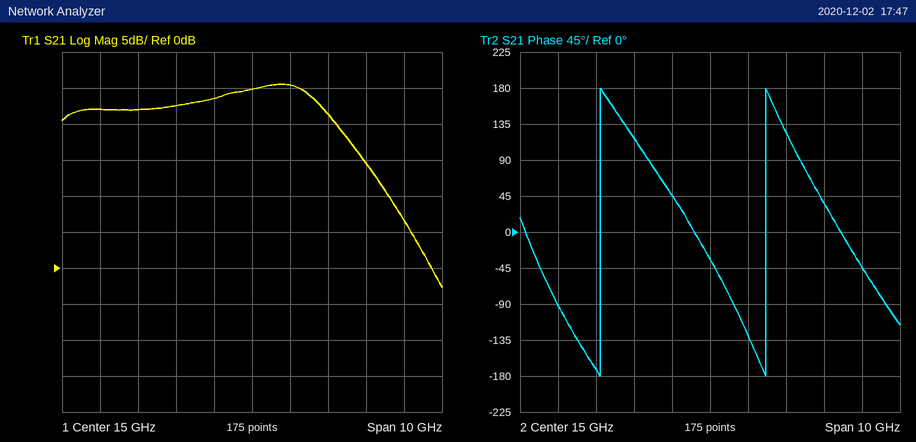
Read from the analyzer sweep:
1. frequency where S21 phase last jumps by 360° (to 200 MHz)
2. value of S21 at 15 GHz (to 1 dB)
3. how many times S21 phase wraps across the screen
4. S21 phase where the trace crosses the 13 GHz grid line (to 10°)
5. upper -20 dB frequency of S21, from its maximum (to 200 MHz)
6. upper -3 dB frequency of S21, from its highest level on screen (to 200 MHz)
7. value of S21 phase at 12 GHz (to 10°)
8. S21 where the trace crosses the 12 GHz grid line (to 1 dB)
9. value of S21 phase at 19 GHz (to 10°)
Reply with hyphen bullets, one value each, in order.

- 16.4 GHz
- 25 dB
- 2
- 120°
- 19.2 GHz
- 16.8 GHz
- -170°
- 22 dB
- -40°
